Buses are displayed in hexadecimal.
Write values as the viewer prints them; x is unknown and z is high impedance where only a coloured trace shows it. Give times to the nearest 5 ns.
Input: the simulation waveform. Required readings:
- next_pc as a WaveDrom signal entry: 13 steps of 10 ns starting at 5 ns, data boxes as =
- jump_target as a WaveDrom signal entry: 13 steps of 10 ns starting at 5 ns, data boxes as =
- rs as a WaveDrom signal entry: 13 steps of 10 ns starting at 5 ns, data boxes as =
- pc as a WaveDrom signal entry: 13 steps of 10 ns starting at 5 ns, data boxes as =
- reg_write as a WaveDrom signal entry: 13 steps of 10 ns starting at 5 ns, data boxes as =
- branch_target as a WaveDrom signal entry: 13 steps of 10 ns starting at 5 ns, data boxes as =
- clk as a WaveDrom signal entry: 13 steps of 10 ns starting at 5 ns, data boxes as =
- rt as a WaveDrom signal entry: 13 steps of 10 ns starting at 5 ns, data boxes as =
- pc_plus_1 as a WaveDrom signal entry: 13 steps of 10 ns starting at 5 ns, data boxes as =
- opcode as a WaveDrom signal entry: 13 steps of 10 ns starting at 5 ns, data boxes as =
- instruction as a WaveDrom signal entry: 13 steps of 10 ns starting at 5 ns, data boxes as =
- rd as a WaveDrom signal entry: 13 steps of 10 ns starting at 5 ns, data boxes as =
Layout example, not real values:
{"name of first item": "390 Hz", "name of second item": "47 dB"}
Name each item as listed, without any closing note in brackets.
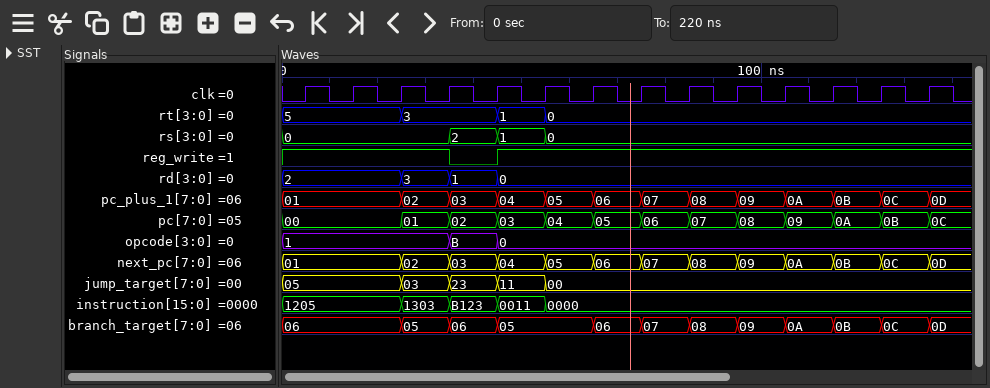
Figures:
{"next_pc as a WaveDrom signal entry: 13 steps of 10 ns starting at 5 ns, data boxes as =": "{name: 'next_pc', wave: '=.===========', data: '01 02 03 04 05 06 07 08 09 0A 0B 0C'}", "jump_target as a WaveDrom signal entry: 13 steps of 10 ns starting at 5 ns, data boxes as =": "{name: 'jump_target', wave: '=.====.......', data: '05 03 23 11 00'}", "rs as a WaveDrom signal entry: 13 steps of 10 ns starting at 5 ns, data boxes as =": "{name: 'rs', wave: '=..===.......', data: '0 2 1 0'}", "pc as a WaveDrom signal entry: 13 steps of 10 ns starting at 5 ns, data boxes as =": "{name: 'pc', wave: '=.===========', data: '00 01 02 03 04 05 06 07 08 09 0A 0B'}", "reg_write as a WaveDrom signal entry: 13 steps of 10 ns starting at 5 ns, data boxes as =": "{name: 'reg_write', wave: '1..01........'}", "branch_target as a WaveDrom signal entry: 13 steps of 10 ns starting at 5 ns, data boxes as =": "{name: 'branch_target', wave: '=.===.=======', data: '06 05 06 05 06 07 08 09 0A 0B 0C'}", "clk as a WaveDrom signal entry: 13 steps of 10 ns starting at 5 ns, data boxes as =": "{name: 'clk', wave: 'p............'}", "rt as a WaveDrom signal entry: 13 steps of 10 ns starting at 5 ns, data boxes as =": "{name: 'rt', wave: '=.=.==.......', data: '5 3 1 0'}", "pc_plus_1 as a WaveDrom signal entry: 13 steps of 10 ns starting at 5 ns, data boxes as =": "{name: 'pc_plus_1', wave: '=.===========', data: '01 02 03 04 05 06 07 08 09 0A 0B 0C'}", "opcode as a WaveDrom signal entry: 13 steps of 10 ns starting at 5 ns, data boxes as =": "{name: 'opcode', wave: '=..==........', data: '1 B 0'}", "instruction as a WaveDrom signal entry: 13 steps of 10 ns starting at 5 ns, data boxes as =": "{name: 'instruction', wave: '=.====.......', data: '1205 1303 B123 0011 0000'}", "rd as a WaveDrom signal entry: 13 steps of 10 ns starting at 5 ns, data boxes as =": "{name: 'rd', wave: '=.===........', data: '2 3 1 0'}"}
